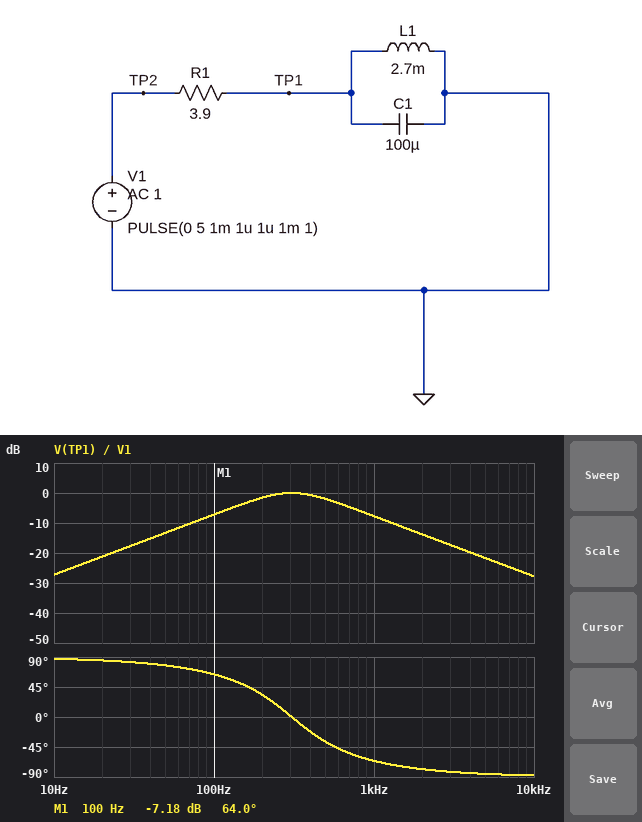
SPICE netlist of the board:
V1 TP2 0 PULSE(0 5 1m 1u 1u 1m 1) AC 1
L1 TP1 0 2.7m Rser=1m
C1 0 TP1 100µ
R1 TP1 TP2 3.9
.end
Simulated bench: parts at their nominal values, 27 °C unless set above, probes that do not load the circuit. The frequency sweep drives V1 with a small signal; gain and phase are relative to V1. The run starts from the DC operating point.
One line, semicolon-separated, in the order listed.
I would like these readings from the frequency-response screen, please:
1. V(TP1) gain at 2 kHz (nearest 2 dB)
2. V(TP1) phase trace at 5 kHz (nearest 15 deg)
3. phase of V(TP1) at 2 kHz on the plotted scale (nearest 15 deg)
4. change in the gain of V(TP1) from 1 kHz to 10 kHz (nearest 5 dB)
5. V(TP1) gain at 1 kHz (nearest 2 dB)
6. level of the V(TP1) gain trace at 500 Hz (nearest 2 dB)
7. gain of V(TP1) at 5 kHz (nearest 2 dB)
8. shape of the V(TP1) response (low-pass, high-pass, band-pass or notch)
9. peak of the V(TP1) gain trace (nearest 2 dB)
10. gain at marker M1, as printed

-14 dB; -90 deg; -75 deg; -20 dB; -8 dB; -2 dB; -22 dB; band-pass; 0 dB; -7.18 dB
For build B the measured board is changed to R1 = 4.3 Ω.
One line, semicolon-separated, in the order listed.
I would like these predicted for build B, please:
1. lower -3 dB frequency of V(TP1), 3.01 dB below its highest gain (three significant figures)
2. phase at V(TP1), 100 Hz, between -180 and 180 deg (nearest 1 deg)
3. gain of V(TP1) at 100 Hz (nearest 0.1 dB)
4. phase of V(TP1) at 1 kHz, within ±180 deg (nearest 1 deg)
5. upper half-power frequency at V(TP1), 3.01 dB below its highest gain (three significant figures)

173 Hz; 66 deg; -7.9 dB; -68 deg; 543 Hz
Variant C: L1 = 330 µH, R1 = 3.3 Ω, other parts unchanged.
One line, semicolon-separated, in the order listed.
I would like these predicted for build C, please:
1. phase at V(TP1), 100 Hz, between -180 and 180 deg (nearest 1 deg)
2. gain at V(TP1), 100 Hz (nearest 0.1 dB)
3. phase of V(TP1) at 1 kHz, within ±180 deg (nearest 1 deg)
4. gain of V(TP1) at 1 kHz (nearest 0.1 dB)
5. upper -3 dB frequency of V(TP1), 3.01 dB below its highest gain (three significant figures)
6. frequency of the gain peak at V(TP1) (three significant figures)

86 deg; -23.9 dB; -26 deg; -0.9 dB; 1.15 kHz; 876 Hz
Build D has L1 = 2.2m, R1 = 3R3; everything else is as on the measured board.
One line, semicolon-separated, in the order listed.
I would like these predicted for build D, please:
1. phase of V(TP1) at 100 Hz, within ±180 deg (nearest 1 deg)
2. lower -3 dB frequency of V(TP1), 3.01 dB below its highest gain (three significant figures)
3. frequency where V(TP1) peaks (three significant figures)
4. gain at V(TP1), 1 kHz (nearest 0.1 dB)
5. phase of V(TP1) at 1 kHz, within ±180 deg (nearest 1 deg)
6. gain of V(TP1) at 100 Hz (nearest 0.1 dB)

65 deg; 175 Hz; 339 Hz; -6.4 dB; -61 deg; -7.6 dB
